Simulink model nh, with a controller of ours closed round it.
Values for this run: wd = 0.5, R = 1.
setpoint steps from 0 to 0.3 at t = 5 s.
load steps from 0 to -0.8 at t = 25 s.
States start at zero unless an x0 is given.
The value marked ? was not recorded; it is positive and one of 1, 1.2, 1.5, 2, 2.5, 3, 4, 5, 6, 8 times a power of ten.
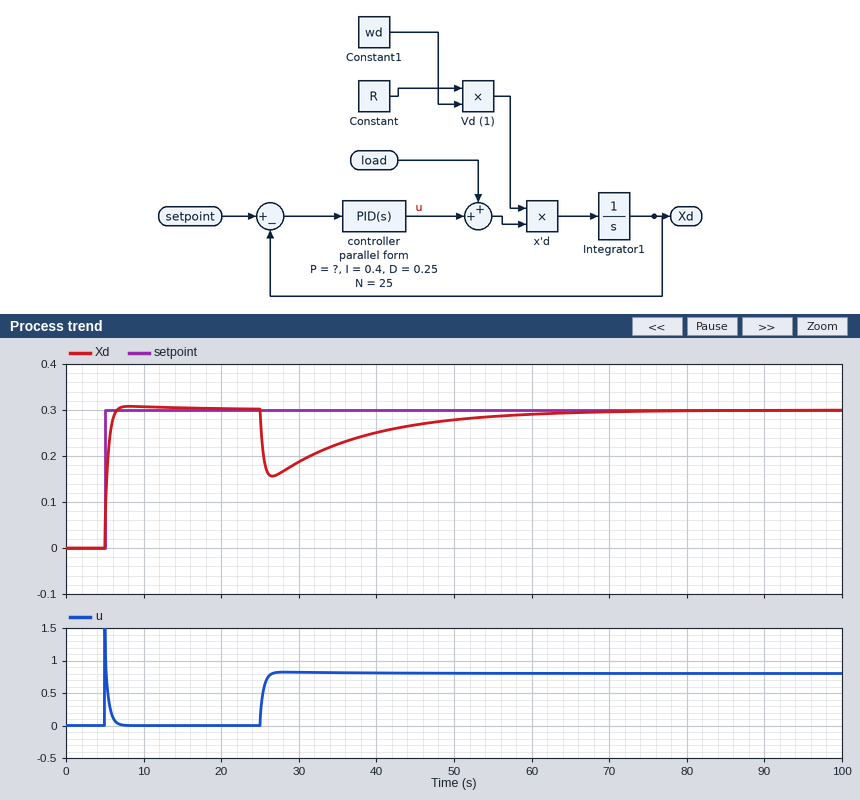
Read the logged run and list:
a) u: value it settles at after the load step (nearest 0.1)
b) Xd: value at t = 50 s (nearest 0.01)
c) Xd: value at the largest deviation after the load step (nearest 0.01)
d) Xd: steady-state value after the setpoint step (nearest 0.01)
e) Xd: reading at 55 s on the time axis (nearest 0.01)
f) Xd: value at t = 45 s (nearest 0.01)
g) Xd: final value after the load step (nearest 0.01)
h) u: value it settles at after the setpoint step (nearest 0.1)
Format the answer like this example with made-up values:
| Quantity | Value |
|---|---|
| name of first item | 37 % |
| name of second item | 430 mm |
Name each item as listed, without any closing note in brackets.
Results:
| Quantity | Value |
|---|---|
| u: value it settles at after the load step | 0.8 |
| Xd: value at t = 50 s | 0.28 |
| Xd: value at the largest deviation after the load step | 0.16 |
| Xd: steady-state value after the setpoint step | 0.30 |
| Xd: reading at 55 s on the time axis | 0.29 |
| Xd: value at t = 45 s | 0.27 |
| Xd: final value after the load step | 0.30 |
| u: value it settles at after the setpoint step | 0.0 |
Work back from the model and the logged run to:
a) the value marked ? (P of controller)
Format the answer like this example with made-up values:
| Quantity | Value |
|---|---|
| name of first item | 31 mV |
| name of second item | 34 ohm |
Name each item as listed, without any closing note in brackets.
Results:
| Quantity | Value |
|---|---|
| the value marked ? | 5 |
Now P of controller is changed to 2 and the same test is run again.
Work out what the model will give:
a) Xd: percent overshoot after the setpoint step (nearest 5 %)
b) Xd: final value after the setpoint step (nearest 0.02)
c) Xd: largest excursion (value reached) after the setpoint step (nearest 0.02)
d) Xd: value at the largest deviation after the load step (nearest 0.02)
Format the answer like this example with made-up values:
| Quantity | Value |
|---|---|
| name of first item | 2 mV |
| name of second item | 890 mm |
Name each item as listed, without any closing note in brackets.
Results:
| Quantity | Value |
|---|---|
| Xd: percent overshoot after the setpoint step | 10 % |
| Xd: final value after the setpoint step | 0.30 |
| Xd: largest excursion (value reached) after the setpoint step | 0.34 |
| Xd: value at the largest deviation after the load step | 0.00 |
